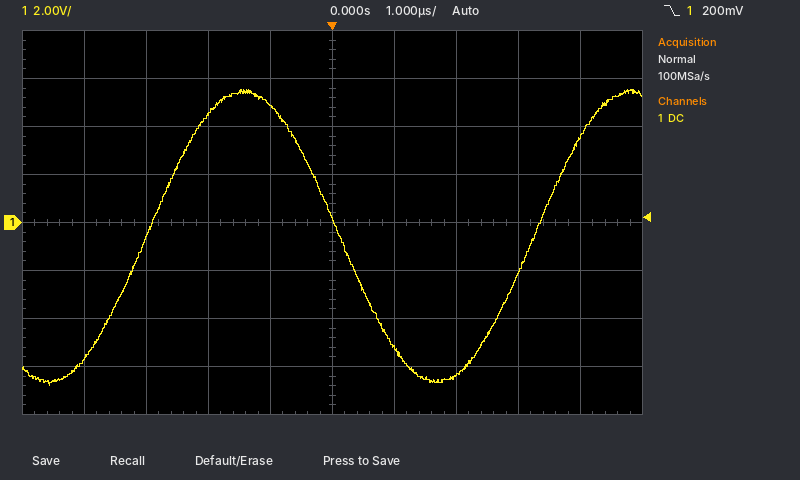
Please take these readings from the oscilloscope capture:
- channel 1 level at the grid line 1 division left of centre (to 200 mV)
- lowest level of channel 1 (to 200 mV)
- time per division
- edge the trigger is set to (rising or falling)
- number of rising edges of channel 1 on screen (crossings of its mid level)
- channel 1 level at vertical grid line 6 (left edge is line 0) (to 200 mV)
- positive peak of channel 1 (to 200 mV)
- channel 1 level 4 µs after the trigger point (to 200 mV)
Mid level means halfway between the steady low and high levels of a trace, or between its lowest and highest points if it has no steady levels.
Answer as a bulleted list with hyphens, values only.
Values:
- 4.8 V
- -6.8 V
- 1 µs
- falling
- 2
- -5.2 V
- 5.6 V
- 3.6 V
